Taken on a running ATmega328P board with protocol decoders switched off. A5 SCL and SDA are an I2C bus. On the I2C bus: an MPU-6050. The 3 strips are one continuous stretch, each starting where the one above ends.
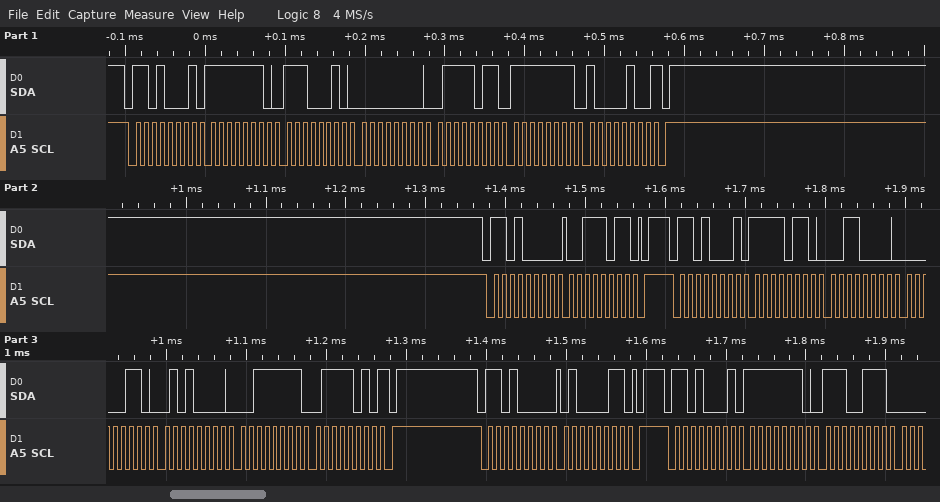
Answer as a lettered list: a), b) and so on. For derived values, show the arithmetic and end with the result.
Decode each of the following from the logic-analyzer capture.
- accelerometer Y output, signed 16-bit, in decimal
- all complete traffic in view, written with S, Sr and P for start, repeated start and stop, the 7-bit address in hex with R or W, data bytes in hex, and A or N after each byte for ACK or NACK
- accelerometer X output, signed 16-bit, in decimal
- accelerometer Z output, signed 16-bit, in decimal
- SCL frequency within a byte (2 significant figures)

a) 0x0650 = 1616
b) S 68R A FE A E2 A 00 A 7B A FF A 84 N P S 68W A 3B A P S 68R A F6 A 30 A 06 A 50 A 3F A 7A N P S 68W A 43 A P S 68R A FE A E7 A
c) 0xF630 = -2512
d) 0x3F7A = 16250
e) 100 kHz
